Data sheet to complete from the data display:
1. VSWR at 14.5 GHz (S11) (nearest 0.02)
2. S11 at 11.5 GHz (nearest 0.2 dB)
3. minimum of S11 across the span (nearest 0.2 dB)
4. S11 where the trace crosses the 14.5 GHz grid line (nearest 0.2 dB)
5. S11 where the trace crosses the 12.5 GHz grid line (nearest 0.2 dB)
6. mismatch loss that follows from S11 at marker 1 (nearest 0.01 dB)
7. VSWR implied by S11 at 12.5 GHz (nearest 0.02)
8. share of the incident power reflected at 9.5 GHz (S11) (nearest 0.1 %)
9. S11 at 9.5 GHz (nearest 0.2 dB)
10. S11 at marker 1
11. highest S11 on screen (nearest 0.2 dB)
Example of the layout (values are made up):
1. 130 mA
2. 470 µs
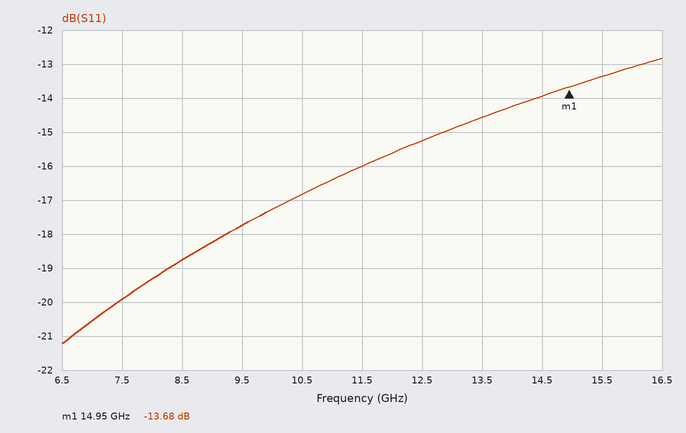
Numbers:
1. 1.50
2. -16.0 dB
3. -21.2 dB
4. -14.0 dB
5. -15.2 dB
6. 0.19 dB
7. 1.42
8. 1.7 %
9. -17.8 dB
10. -13.68 dB
11. -12.8 dB
